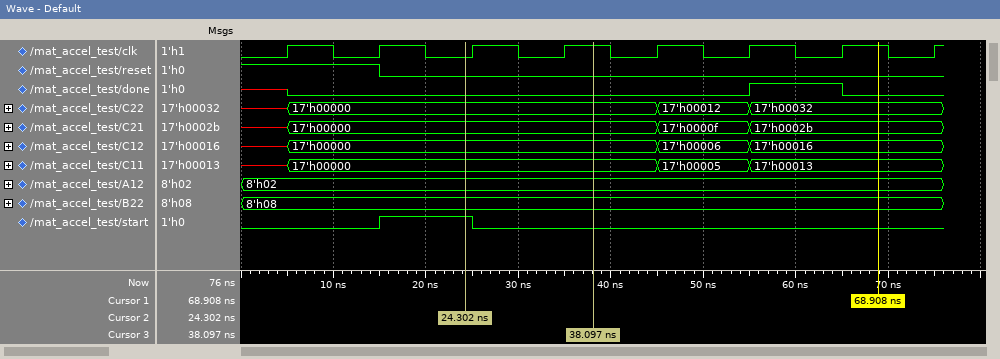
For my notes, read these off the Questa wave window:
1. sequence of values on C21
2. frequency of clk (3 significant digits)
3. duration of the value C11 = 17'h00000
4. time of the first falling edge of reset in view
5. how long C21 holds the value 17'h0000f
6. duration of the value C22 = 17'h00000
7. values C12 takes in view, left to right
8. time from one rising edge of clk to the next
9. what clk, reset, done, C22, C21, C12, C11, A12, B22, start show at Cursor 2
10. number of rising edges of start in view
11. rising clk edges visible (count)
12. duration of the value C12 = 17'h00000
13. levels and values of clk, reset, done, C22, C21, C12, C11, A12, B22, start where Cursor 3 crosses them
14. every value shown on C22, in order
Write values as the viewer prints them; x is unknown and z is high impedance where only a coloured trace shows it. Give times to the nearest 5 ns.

x, 17'h00000, 17'h0000f, 17'h0002b
100 MHz
40 ns
15 ns
10 ns
40 ns
x, 17'h00000, 17'h00006, 17'h00016
10 ns
clk=0, reset=0, done=0, C22=17'h00000, C21=17'h00000, C12=17'h00000, C11=17'h00000, A12=8'h02, B22=8'h08, start=1
1
8
40 ns
clk=1, reset=0, done=0, C22=17'h00000, C21=17'h00000, C12=17'h00000, C11=17'h00000, A12=8'h02, B22=8'h08, start=0
x, 17'h00000, 17'h00012, 17'h00032
